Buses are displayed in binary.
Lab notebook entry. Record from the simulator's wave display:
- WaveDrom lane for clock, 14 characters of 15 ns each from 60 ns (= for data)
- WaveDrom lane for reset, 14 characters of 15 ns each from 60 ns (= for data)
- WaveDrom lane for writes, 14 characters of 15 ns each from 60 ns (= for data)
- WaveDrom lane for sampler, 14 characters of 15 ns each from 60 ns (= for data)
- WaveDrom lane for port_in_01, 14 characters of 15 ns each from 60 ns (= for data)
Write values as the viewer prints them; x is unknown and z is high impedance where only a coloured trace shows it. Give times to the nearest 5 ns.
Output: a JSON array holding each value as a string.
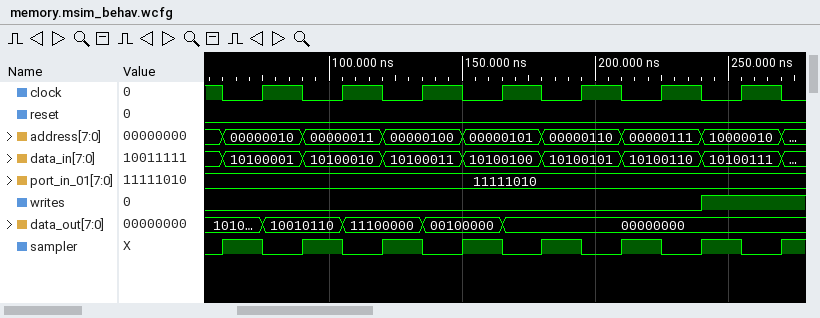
["{name: 'clock', wave: '01010101010101'}", "{name: 'reset', wave: '0.............'}", "{name: 'writes', wave: '0...........1.'}", "{name: 'sampler', wave: '10101010101010'}", "{name: 'port_in_01', wave: '=.............', data: '11111010'}"]
